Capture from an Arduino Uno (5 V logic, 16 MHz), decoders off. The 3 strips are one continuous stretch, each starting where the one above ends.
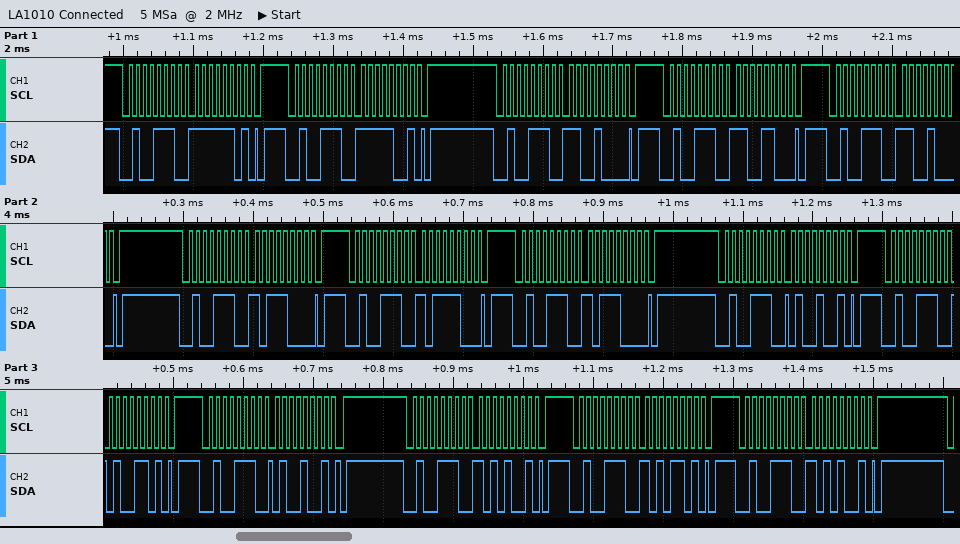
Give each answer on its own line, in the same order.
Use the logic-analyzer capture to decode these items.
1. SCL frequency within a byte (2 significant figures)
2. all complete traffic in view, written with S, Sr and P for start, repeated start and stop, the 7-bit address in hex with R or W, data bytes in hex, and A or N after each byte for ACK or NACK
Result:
100 kHz
S 27W A FD A P S 27W A F9 A P S 27W A C8 A P S 27W A CC A P S 27W A C8 A P S 27W A B8 A P S 27W A BC A P S 27W A B8 A P S 27W A 49 A P S 27W A 4D A P S 27W A 49 A P S 27W A A9 A P S 27W A AD A P S 27W A A9 A P
